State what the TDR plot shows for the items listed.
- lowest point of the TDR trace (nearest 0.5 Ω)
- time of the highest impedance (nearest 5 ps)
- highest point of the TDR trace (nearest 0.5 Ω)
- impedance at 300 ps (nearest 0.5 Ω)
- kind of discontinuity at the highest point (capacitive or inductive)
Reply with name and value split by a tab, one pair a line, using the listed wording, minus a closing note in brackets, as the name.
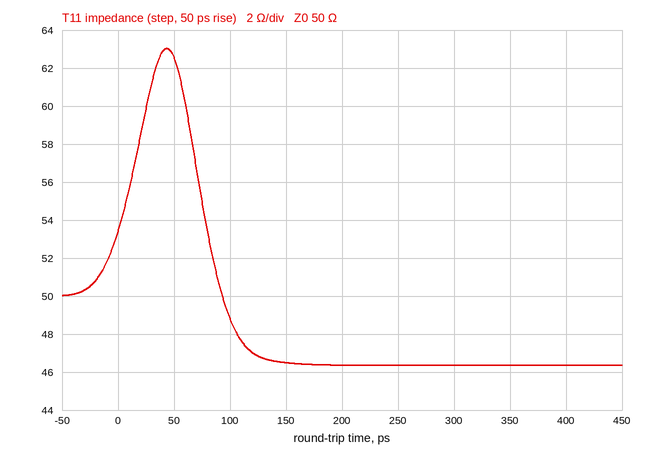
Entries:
lowest point of the TDR trace	46.5 Ω
time of the highest impedance	45 ps
highest point of the TDR trace	63.0 Ω
impedance at 300 ps	46.5 Ω
kind of discontinuity at the highest point	inductive
